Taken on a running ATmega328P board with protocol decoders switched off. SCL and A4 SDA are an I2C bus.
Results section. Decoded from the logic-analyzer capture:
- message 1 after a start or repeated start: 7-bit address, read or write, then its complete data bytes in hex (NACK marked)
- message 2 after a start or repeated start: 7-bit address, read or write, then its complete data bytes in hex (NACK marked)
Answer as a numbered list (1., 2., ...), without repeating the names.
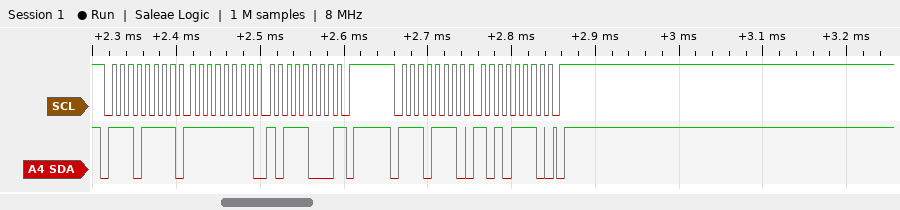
1. 0x77 read: FF B8 NACK
2. 0x77 write: AE
